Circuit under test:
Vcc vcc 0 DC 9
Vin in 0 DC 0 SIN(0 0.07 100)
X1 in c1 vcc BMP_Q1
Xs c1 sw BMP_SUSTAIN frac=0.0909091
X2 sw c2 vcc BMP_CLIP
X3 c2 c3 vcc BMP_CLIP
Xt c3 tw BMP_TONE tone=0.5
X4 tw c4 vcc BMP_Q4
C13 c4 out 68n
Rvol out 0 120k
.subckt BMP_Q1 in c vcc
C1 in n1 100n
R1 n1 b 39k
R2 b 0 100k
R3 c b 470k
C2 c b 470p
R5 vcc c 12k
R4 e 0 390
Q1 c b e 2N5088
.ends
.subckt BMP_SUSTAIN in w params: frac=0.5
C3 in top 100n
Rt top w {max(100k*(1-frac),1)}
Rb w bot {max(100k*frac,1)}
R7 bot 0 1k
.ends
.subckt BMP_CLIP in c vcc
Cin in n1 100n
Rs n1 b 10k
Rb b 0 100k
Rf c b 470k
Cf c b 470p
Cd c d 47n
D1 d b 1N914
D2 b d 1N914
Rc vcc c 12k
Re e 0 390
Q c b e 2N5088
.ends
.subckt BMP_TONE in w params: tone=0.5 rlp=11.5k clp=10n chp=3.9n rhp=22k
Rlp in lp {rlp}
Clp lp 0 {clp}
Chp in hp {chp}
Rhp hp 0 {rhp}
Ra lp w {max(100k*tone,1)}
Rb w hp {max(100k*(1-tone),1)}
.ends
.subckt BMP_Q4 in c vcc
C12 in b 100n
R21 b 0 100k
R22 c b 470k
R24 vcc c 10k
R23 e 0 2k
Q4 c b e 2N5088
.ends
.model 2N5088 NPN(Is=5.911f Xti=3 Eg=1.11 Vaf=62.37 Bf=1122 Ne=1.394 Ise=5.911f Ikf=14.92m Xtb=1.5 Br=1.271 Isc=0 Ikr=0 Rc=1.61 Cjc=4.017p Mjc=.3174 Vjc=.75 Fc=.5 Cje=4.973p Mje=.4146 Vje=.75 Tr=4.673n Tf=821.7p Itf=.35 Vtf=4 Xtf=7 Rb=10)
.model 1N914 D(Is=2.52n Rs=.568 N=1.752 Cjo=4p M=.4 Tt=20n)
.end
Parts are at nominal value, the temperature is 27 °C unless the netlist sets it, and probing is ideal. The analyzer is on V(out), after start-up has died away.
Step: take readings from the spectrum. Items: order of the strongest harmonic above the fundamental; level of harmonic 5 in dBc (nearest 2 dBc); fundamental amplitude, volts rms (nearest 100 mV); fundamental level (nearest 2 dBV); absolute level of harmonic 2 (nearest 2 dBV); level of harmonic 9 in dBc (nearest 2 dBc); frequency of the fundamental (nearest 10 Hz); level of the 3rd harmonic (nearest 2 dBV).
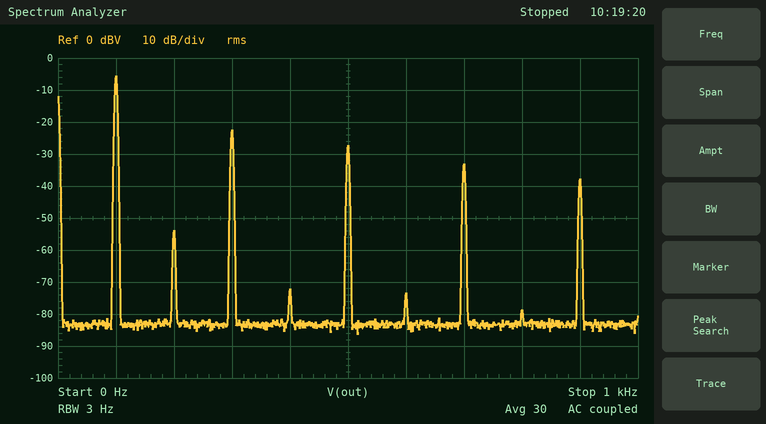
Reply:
3
-22 dBc
500 mV
-6 dBV
-54 dBV
-32 dBc
100 Hz
-22 dBV
